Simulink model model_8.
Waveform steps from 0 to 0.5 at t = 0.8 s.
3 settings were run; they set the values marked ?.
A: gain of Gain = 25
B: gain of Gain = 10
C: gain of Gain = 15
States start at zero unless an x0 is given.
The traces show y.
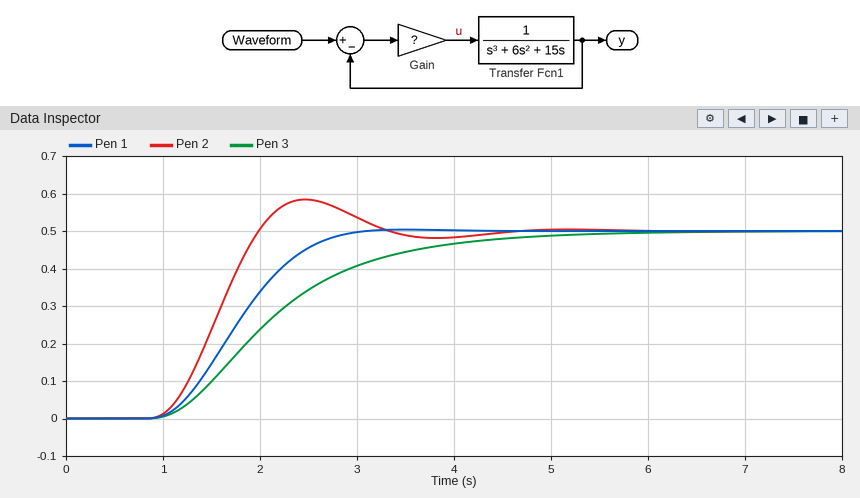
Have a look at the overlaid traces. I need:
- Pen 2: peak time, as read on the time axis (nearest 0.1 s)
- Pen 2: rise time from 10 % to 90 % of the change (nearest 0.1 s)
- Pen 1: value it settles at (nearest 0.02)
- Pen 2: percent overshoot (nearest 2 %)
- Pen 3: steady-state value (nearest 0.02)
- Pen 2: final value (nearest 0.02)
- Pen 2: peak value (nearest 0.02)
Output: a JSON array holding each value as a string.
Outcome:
["2.5 s", "0.7 s", "0.50", "16 %", "0.50", "0.50", "0.58"]
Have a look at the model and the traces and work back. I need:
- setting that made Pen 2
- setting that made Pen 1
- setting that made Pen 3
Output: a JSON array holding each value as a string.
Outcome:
["A", "C", "B"]
